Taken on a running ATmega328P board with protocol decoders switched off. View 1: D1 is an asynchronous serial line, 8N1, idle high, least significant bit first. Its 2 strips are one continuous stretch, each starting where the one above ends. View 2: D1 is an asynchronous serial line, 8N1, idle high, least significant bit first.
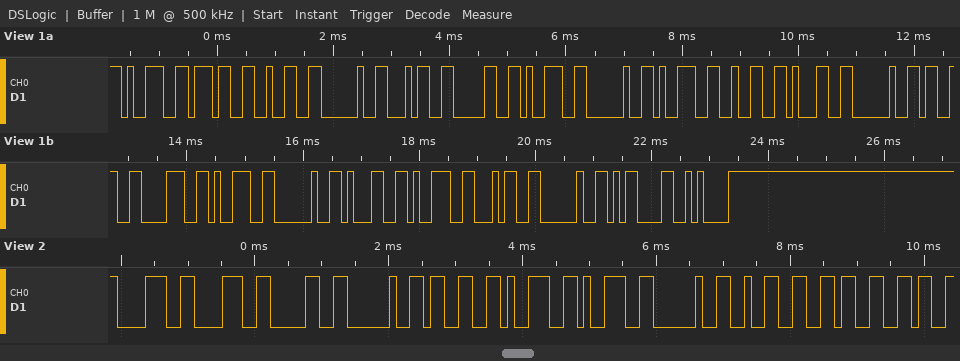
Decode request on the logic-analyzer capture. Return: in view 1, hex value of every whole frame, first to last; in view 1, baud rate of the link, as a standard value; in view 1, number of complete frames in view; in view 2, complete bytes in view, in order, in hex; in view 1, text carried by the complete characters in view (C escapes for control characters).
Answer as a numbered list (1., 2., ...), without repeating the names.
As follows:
1. 39 37 32 20 34 30 39 20 39 32 31 20 33 38 39 20 31 39 34 20 0D 0A
2. 9600 baud
3. 22
4. 38 38 30 20 33 39 39 20 32 36 36
5. "972 409 921 389 194 \r\n"
